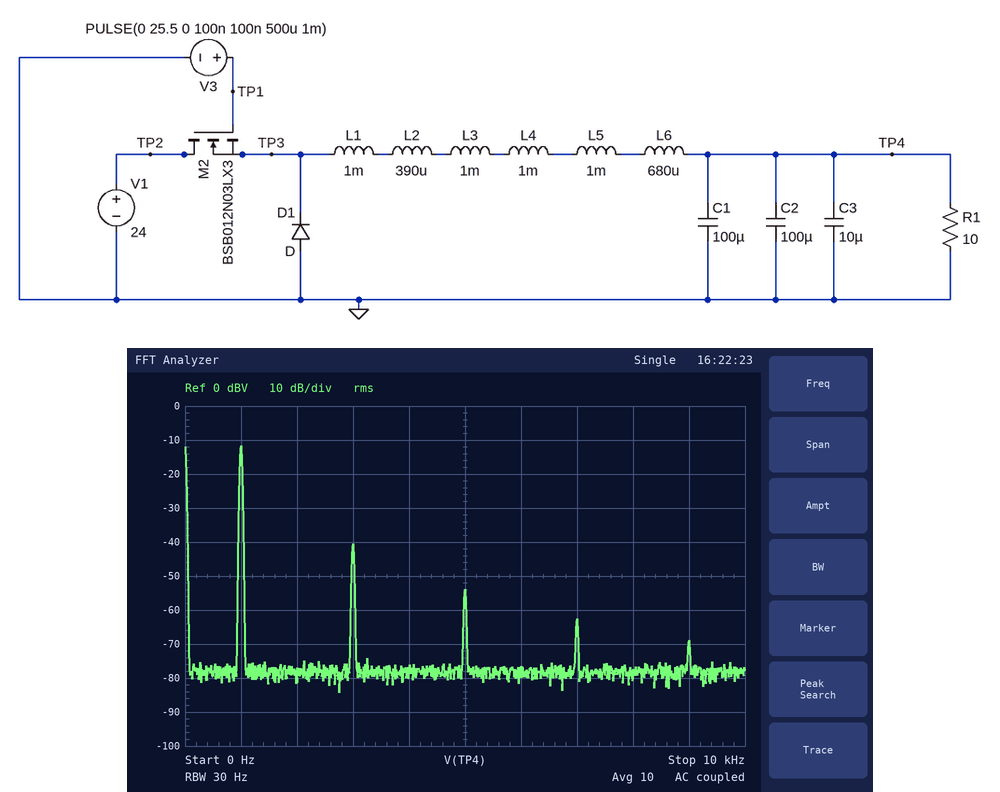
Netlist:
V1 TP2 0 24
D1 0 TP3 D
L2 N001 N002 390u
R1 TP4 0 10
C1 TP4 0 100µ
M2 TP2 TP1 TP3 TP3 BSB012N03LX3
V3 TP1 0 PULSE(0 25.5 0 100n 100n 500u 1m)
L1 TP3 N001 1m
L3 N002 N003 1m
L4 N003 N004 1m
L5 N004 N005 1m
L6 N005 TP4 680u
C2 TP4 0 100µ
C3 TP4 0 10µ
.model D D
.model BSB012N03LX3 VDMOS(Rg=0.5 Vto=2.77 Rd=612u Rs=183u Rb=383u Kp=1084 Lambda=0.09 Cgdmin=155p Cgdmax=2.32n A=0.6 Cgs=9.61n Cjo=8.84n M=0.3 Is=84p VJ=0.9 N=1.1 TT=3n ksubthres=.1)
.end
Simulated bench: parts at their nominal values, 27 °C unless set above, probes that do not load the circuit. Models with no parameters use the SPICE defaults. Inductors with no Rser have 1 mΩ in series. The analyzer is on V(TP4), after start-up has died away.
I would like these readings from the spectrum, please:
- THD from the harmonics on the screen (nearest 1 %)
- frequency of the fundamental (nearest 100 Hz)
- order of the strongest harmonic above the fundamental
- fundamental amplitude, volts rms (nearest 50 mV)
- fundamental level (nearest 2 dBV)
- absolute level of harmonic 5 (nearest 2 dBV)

4 %
1.0 kHz
3
250 mV
-12 dBV
-54 dBV
